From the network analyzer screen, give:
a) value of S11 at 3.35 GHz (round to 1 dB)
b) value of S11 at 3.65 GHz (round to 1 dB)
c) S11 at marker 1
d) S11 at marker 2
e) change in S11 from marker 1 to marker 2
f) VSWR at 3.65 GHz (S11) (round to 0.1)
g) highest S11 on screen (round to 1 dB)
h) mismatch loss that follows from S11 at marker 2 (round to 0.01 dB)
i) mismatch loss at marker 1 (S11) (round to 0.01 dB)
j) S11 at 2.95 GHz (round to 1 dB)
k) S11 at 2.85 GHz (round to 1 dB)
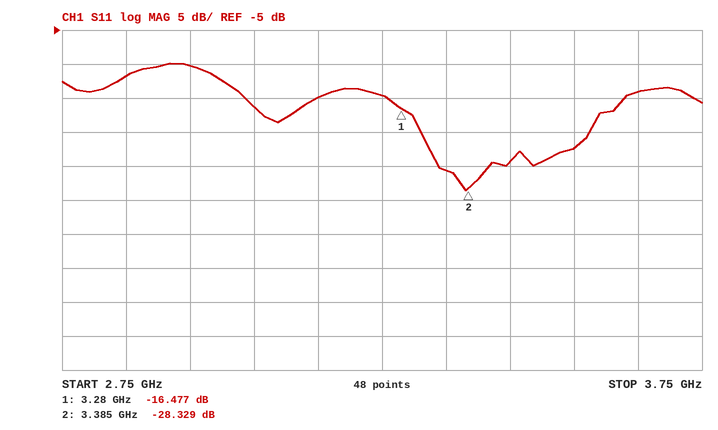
-26 dB
-14 dB
-16.477 dB
-28.329 dB
-11.852 dB
1.5
-10 dB
0.01 dB
0.10 dB
-10 dB
-12 dB
